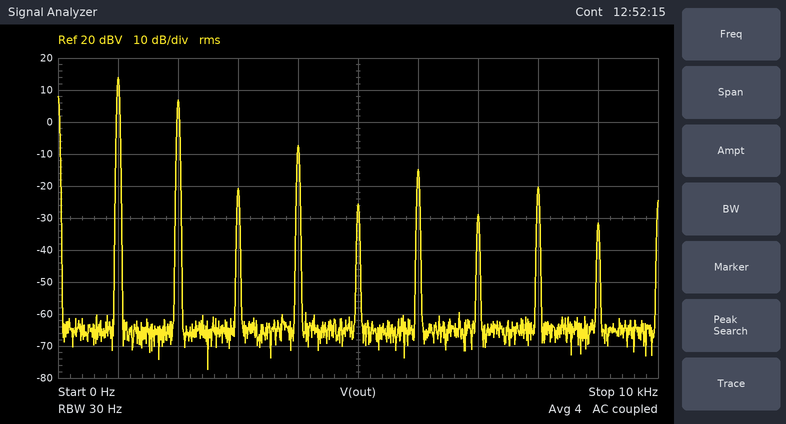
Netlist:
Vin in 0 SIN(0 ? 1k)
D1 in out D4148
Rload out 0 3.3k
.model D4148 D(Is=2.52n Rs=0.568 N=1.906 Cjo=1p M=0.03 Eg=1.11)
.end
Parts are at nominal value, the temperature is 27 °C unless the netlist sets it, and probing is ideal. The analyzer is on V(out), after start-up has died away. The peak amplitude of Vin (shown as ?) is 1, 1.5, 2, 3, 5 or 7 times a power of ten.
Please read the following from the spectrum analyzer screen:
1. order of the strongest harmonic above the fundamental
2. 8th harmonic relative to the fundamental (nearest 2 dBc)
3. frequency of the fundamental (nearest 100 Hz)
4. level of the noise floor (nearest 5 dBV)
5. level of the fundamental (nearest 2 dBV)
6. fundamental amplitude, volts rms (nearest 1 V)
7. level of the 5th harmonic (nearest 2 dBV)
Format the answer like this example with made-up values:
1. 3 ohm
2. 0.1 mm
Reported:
1. 2
2. -34 dBc
3. 1.0 kHz
4. -65 dBV
5. 14 dBV
6. 5 V
7. -26 dBV
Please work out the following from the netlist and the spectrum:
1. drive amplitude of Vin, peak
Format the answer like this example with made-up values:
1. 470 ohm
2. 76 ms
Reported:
1. 15 V
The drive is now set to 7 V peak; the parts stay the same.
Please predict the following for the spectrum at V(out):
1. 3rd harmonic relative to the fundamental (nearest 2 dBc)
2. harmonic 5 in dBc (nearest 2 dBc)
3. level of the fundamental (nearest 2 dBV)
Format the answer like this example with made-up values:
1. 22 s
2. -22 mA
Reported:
1. -28 dBc
2. -34 dBc
3. 6 dBV
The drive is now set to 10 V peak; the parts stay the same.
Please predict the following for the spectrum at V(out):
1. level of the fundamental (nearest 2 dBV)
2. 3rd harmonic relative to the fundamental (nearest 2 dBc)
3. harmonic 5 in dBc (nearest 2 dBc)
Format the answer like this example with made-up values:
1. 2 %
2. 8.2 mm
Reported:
1. 10 dBV
2. -32 dBc
3. -36 dBc
